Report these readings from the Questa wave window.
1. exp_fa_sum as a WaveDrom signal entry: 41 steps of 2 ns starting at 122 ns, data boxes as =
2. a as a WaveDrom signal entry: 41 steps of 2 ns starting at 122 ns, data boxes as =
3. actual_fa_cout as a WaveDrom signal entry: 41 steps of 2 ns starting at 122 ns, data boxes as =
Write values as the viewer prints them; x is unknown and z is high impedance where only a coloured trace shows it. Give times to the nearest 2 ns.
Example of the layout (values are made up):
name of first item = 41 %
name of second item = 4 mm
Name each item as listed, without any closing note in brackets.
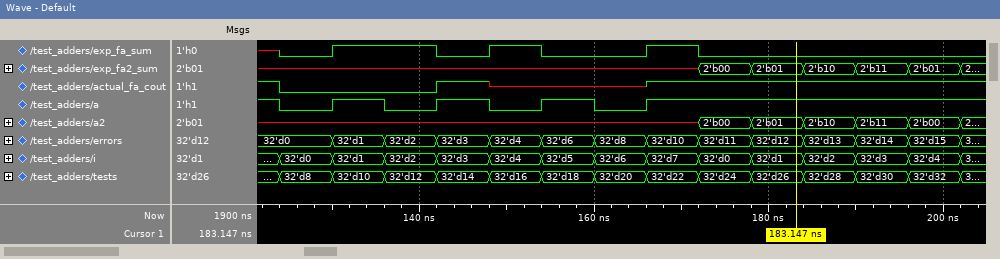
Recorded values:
exp_fa_sum as a WaveDrom signal entry: 41 steps of 2 ns starting at 122 ns, data boxes as = = {name: 'exp_fa_sum', wave: 'x0..1.....0..1..0.....1..0...............'}
a as a WaveDrom signal entry: 41 steps of 2 ns starting at 122 ns, data boxes as = = {name: 'a', wave: '10..1..0..1..0..1..0..1..................'}
actual_fa_cout as a WaveDrom signal entry: 41 steps of 2 ns starting at 122 ns, data boxes as = = {name: 'actual_fa_cout', wave: '10........1..x........1..................'}
